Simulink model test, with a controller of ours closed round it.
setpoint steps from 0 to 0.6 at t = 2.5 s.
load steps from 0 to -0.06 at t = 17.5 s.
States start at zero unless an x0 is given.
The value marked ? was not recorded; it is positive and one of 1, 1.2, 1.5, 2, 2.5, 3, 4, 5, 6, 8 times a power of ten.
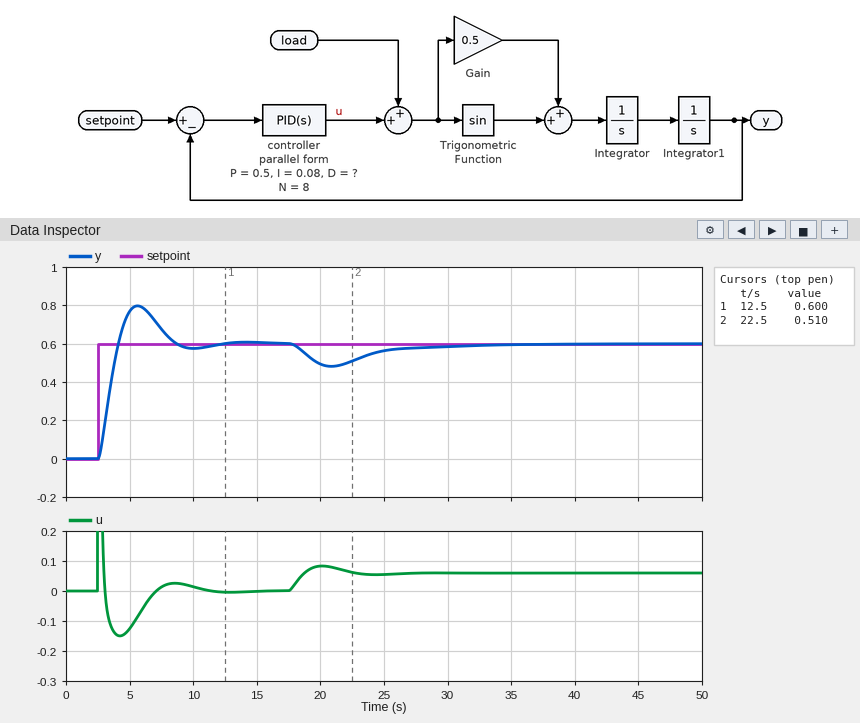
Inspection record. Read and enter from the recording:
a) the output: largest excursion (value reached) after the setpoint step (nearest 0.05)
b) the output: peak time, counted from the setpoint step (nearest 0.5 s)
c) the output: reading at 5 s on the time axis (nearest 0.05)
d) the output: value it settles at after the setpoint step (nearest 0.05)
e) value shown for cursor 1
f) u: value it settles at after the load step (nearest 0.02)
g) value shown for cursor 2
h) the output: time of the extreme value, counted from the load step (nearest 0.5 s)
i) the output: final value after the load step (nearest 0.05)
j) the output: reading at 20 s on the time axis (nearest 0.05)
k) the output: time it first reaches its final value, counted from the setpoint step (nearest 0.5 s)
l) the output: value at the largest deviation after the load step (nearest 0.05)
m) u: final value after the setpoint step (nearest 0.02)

0.80
3.0 s
0.75
0.60
0.600
0.06
0.510
3.5 s
0.60
0.50
1.5 s
0.50
0.00
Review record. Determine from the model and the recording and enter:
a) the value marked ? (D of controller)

0.6
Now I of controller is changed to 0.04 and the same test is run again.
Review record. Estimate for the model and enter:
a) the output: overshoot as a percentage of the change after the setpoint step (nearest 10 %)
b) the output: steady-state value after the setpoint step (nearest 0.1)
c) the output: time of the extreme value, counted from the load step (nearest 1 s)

30 %
0.6
4 s
